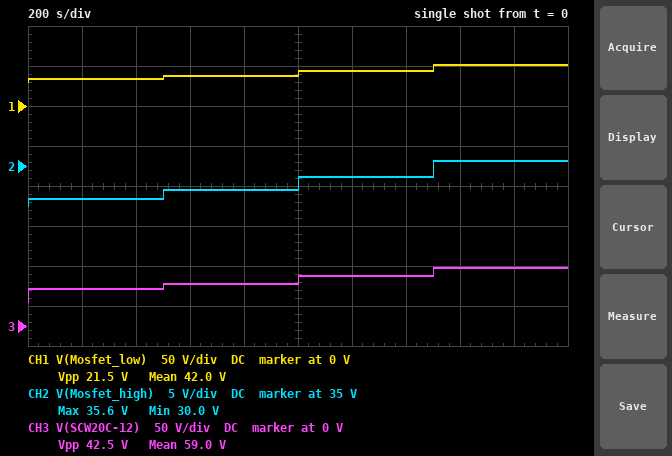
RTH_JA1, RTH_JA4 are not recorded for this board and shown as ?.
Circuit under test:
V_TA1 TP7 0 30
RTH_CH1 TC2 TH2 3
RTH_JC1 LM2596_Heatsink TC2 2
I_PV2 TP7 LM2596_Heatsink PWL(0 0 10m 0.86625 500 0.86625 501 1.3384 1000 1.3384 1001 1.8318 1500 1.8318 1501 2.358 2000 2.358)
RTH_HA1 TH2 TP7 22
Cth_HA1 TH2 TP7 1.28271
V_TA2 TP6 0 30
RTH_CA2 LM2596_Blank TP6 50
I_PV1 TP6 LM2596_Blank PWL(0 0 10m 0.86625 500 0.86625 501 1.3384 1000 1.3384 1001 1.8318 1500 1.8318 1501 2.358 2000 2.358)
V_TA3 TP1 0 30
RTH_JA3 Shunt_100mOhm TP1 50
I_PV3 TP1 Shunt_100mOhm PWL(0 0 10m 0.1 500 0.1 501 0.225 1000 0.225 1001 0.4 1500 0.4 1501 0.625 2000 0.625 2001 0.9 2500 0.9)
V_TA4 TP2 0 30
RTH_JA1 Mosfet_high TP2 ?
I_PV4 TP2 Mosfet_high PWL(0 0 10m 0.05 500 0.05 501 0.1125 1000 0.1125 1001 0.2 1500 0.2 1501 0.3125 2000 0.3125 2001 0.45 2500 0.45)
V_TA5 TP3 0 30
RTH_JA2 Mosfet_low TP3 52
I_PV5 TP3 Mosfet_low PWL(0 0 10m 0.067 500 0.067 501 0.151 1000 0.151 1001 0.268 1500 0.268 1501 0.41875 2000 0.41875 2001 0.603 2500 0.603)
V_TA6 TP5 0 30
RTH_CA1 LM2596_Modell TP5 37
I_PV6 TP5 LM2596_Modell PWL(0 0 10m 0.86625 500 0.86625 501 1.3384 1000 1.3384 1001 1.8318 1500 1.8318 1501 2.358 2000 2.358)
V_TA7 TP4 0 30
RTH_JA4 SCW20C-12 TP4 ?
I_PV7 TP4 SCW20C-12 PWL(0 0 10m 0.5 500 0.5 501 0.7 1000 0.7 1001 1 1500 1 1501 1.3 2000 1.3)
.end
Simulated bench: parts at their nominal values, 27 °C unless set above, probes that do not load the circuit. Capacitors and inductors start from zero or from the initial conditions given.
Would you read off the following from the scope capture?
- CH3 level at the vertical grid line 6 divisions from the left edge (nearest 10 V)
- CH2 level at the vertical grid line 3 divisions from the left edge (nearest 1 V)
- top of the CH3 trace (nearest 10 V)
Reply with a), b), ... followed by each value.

a) 60 V
b) 32 V
c) 70 V
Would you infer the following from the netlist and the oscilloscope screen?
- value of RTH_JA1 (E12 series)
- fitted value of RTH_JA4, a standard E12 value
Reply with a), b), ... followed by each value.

a) 18 Ω
b) 33 Ω
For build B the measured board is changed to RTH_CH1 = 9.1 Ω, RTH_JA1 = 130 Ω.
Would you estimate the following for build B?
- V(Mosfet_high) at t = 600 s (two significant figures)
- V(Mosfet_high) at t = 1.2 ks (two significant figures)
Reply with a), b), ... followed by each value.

a) 45 V
b) 56 V
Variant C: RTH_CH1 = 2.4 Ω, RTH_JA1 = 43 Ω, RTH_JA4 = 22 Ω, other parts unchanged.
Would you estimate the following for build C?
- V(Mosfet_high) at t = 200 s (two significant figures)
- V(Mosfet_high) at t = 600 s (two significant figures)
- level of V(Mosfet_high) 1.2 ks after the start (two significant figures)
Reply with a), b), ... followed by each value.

a) 32 V
b) 35 V
c) 39 V
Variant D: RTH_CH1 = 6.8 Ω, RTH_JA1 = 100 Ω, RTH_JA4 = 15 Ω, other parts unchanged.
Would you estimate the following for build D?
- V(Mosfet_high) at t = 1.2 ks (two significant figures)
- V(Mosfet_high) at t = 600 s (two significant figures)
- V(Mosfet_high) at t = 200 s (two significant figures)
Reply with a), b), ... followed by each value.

a) 50 V
b) 41 V
c) 35 V
